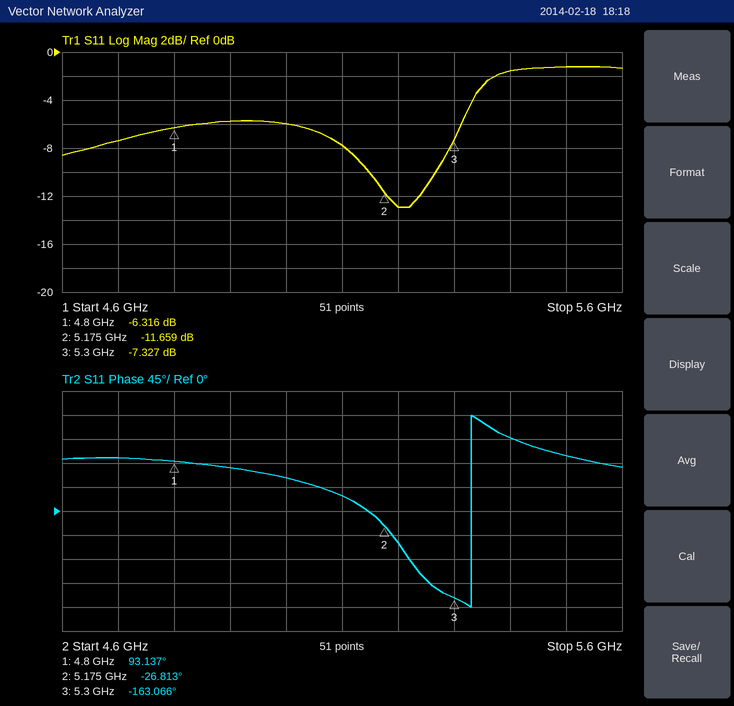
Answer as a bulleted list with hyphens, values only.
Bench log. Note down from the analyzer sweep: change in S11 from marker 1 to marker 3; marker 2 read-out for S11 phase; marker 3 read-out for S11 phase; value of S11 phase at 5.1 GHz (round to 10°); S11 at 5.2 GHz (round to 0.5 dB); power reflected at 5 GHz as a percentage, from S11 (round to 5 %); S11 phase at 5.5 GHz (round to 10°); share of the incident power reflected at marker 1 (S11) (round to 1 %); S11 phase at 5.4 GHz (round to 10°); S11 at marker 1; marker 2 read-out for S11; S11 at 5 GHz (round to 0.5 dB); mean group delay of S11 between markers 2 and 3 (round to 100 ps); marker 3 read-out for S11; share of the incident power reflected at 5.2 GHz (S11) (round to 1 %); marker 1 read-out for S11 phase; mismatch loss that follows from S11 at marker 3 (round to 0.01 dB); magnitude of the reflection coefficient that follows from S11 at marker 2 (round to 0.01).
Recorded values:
- -1.011 dB
- -26.813°
- -163.066°
- 30°
- -13.0 dB
- 25 %
- 100°
- 23 %
- 140°
- -6.316 dB
- -11.659 dB
- -6.0 dB
- 3.0 ns
- -7.327 dB
- 5 %
- 93.137°
- 0.89 dB
- 0.26
